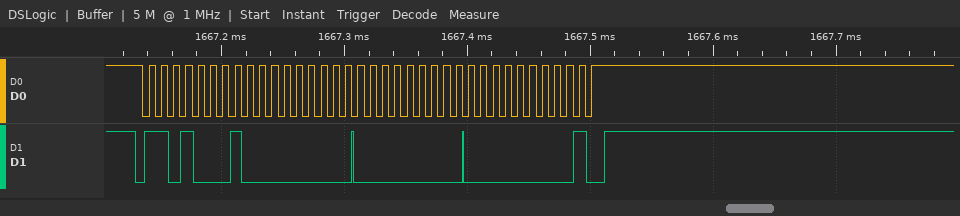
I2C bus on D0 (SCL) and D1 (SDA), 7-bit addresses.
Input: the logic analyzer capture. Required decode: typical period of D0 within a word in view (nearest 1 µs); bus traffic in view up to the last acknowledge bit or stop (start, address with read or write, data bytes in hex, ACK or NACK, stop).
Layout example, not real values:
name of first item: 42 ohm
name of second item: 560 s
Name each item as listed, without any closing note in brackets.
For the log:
typical period of D0 within a word in view: 10 µs
bus traffic in view up to the last acknowledge bit or stop: start, address 68 read ACK, 00 ACK, 00 ACK, 00 NACK, stop
